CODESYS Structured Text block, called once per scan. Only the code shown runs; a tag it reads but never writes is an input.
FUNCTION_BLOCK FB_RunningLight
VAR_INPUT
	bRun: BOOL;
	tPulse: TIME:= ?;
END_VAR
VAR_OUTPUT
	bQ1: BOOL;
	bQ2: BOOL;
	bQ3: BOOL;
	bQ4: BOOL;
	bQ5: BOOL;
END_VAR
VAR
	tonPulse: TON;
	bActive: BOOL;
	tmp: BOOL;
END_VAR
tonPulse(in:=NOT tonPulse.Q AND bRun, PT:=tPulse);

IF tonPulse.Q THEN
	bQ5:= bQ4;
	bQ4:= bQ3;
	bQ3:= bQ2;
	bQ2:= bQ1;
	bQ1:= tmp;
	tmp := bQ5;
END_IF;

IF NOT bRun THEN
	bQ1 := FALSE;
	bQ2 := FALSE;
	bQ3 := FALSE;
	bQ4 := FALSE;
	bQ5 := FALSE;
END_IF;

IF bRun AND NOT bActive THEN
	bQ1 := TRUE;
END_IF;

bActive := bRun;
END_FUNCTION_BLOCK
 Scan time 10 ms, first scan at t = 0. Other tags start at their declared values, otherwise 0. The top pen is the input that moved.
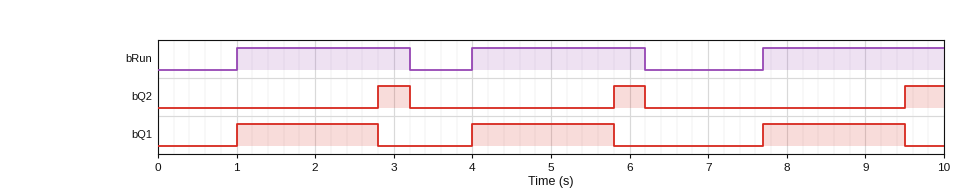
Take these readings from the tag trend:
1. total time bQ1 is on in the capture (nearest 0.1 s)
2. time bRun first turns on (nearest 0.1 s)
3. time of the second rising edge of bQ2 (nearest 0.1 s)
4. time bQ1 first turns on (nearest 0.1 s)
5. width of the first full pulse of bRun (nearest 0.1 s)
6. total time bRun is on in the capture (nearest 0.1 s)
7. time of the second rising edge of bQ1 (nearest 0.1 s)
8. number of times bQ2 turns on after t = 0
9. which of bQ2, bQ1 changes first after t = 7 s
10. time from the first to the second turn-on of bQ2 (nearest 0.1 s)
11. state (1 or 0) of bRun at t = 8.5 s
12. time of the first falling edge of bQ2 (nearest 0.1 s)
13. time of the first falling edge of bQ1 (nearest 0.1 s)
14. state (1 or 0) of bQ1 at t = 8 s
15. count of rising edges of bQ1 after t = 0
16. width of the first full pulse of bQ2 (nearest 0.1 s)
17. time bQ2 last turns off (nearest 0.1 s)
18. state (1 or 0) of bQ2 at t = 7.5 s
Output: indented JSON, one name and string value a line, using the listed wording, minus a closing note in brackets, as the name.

{
  "total time bQ1 is on in the capture": "5.4 s",
  "time bRun first turns on": "1.0 s",
  "time of the second rising edge of bQ2": "5.8 s",
  "time bQ1 first turns on": "1.0 s",
  "width of the first full pulse of bRun": "2.2 s",
  "total time bRun is on in the capture": "6.7 s",
  "time of the second rising edge of bQ1": "4.0 s",
  "number of times bQ2 turns on after t = 0": "3",
  "which of bQ2, bQ1 changes first after t = 7 s": "bQ1",
  "time from the first to the second turn-on of bQ2": "3.0 s",
  "state (1 or 0) of bRun at t = 8.5 s": "1",
  "time of the first falling edge of bQ2": "3.2 s",
  "time of the first falling edge of bQ1": "2.8 s",
  "state (1 or 0) of bQ1 at t = 8 s": "1",
  "count of rising edges of bQ1 after t = 0": "3",
  "width of the first full pulse of bQ2": "0.4 s",
  "time bQ2 last turns off": "6.2 s",
  "state (1 or 0) of bQ2 at t = 7.5 s": "0"
}
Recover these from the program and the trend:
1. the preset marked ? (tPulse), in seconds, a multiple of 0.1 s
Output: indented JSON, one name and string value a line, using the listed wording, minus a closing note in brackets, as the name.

{
  "the preset marked ? (tPulse), in seconds, a multiple of 0.1 s": "1.8 s"
}
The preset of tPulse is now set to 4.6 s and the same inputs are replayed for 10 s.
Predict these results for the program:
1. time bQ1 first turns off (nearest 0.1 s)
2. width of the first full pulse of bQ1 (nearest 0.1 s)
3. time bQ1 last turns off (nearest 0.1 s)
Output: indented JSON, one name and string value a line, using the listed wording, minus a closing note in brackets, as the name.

{
  "time bQ1 first turns off": "3.2 s",
  "width of the first full pulse of bQ1": "2.2 s",
  "time bQ1 last turns off": "6.2 s"
}
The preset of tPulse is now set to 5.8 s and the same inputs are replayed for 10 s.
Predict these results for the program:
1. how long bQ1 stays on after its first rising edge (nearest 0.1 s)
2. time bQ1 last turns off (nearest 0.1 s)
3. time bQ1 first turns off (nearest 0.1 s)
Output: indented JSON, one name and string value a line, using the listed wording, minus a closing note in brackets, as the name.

{
  "how long bQ1 stays on after its first rising edge": "2.2 s",
  "time bQ1 last turns off": "6.2 s",
  "time bQ1 first turns off": "3.2 s"
}
